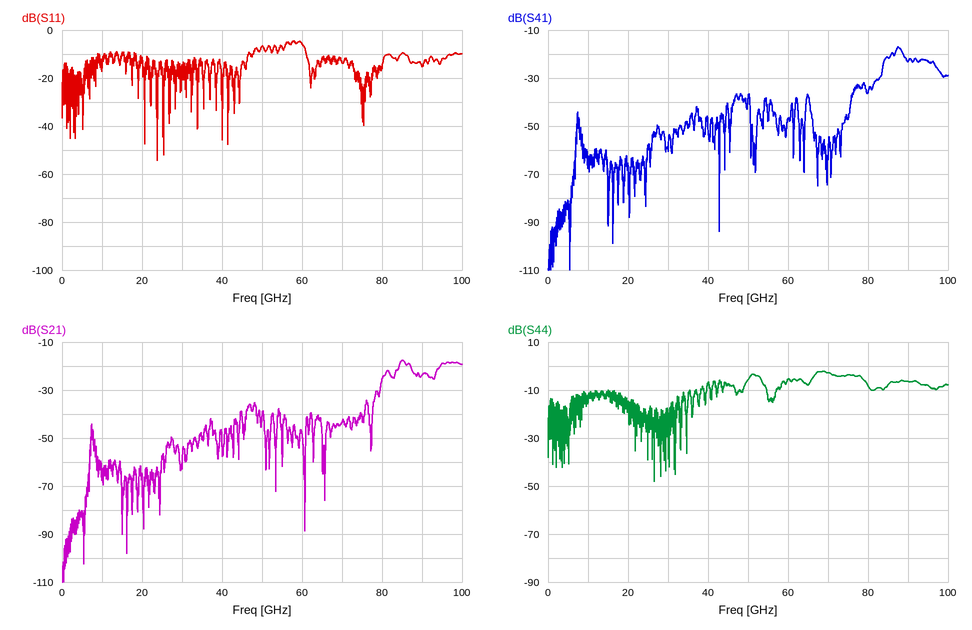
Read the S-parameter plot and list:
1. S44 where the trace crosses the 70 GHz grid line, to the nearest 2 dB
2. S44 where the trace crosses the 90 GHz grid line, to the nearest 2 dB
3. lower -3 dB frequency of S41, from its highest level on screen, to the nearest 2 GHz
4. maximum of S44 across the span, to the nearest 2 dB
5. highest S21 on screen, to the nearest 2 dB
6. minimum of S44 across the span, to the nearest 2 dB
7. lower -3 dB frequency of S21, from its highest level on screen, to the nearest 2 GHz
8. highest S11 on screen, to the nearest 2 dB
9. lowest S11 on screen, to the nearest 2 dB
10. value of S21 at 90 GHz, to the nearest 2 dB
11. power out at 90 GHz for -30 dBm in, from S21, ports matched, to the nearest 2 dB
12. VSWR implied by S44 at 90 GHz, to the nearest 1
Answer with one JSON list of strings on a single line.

["-2 dB", "-6 dB", "86 GHz", "-2 dB", "-18 dB", "-48 dB", "84 GHz", "-4 dB", "-54 dB", "-24 dB", "-54 dBm", "3"]
